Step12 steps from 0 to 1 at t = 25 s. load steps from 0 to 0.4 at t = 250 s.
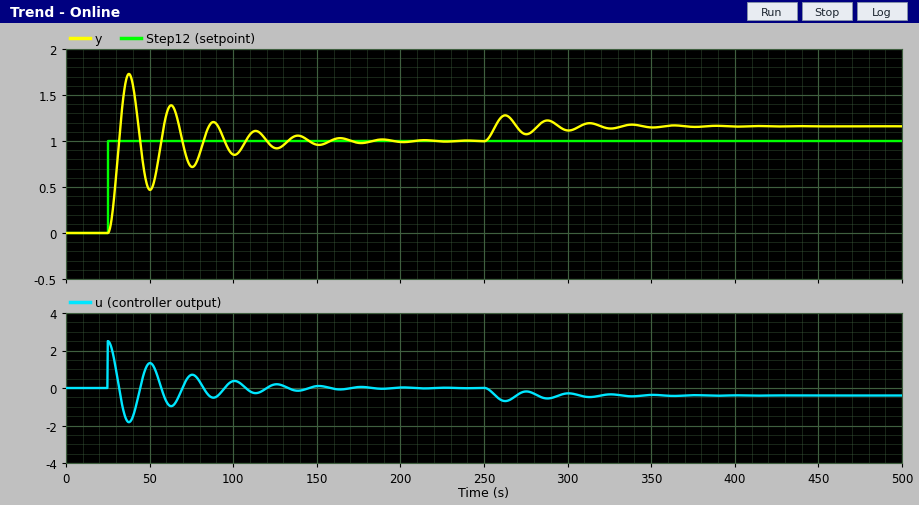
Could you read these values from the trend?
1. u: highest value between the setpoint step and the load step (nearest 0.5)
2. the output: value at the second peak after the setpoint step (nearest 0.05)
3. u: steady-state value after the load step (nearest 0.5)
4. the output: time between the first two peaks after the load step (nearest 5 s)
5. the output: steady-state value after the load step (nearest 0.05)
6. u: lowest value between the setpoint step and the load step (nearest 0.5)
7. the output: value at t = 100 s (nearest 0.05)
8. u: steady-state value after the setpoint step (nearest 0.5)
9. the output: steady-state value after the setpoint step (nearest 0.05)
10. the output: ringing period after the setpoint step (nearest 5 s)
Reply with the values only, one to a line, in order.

2.5
1.40
-0.5
25 s
1.15
-2.0
0.85
0.0
1.00
25 s
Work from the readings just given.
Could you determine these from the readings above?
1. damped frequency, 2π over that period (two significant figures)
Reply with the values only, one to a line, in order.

0.25 rad/s
